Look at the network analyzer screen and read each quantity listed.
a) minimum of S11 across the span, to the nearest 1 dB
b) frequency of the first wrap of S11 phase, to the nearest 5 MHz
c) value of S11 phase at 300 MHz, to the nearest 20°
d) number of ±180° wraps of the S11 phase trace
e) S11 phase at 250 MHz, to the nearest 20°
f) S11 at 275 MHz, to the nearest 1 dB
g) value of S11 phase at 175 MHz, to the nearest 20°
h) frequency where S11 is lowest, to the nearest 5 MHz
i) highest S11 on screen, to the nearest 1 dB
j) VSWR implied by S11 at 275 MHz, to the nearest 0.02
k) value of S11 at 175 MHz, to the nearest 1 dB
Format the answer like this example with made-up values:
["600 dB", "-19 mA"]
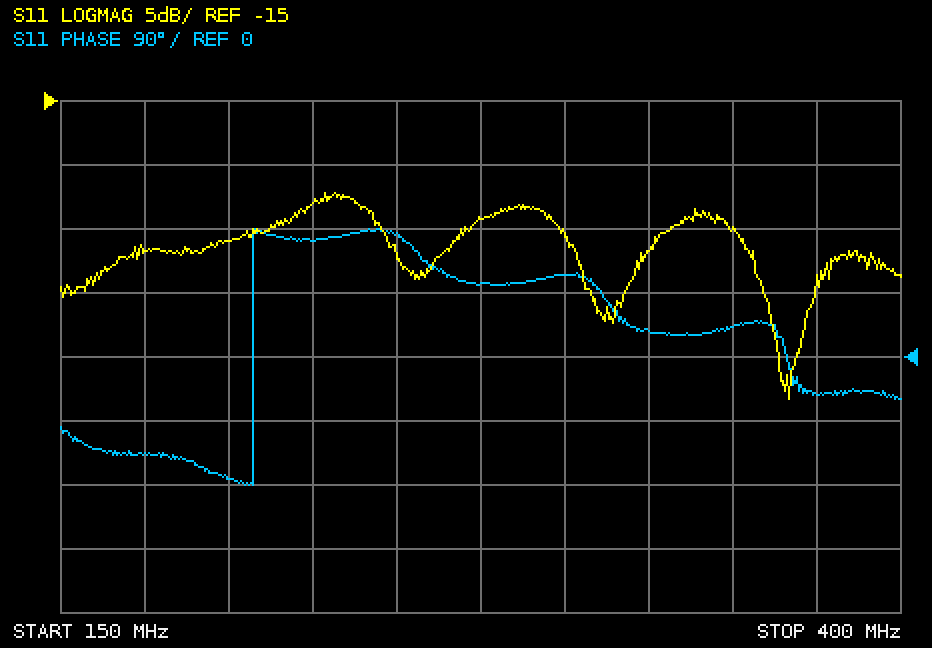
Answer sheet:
["-38 dB", "205 MHz", "120°", "1", "180°", "-24 dB", "-140°", "365 MHz", "-22 dB", "1.14", "-27 dB"]
